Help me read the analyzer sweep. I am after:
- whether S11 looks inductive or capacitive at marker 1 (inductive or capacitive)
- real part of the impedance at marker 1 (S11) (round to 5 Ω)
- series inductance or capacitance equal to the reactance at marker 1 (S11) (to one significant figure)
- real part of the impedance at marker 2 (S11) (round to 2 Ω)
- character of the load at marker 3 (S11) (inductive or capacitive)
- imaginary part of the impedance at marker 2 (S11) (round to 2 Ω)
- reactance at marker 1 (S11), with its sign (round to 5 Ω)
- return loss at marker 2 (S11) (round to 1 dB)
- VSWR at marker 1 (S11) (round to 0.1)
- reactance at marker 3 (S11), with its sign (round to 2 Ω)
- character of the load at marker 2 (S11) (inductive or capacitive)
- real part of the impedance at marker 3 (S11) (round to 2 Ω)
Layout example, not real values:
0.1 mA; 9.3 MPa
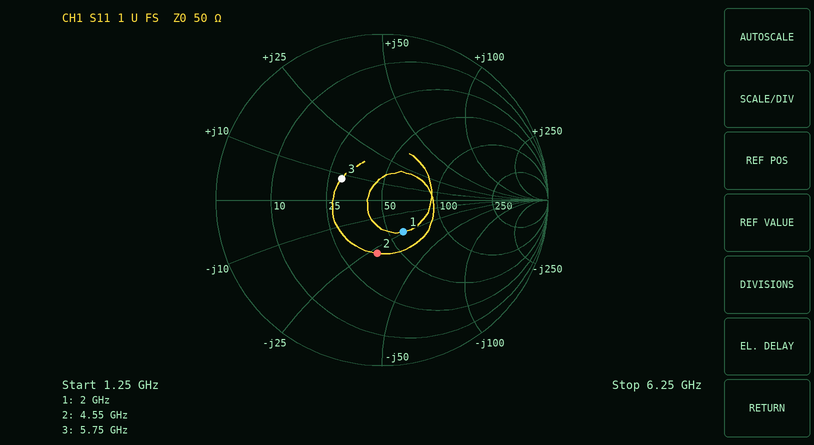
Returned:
capacitive; 60 Ω; 3 pF; 38 Ω; inductive; -28 Ω; -25 Ω; 10 dB; 1.6; +8 Ω; capacitive; 30 Ω
